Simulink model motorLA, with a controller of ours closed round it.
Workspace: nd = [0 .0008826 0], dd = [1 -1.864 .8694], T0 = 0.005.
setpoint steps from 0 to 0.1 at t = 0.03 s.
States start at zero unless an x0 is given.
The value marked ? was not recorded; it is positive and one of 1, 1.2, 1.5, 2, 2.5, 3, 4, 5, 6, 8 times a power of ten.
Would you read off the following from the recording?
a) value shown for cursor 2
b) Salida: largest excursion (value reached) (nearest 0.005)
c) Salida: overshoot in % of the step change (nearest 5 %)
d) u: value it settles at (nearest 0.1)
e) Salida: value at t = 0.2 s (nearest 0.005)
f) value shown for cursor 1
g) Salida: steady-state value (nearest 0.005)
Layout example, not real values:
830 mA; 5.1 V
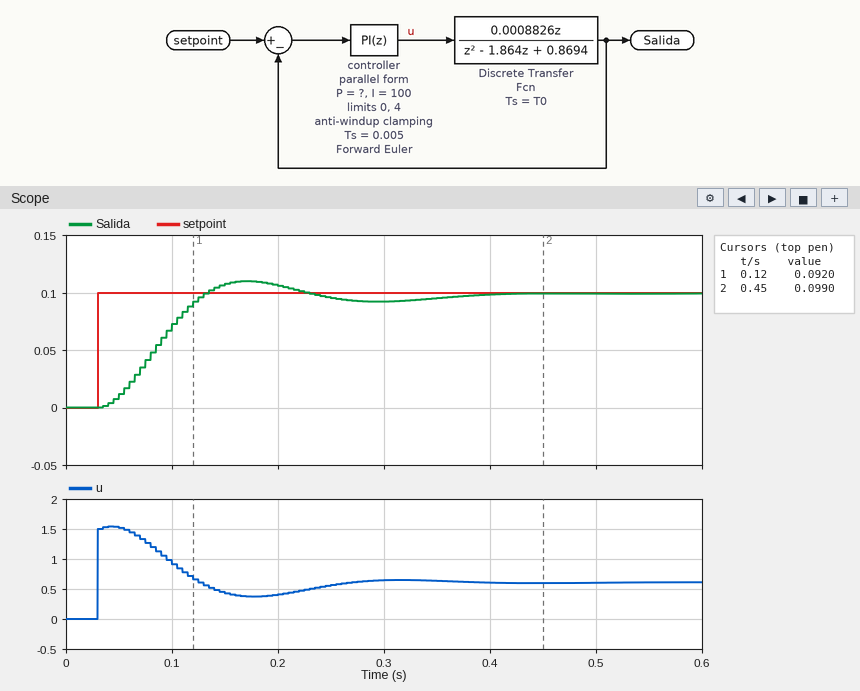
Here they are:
0.0990; 0.110; 10 %; 0.6; 0.105; 0.0920; 0.100
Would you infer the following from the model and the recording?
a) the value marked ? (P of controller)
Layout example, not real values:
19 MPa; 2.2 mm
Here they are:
15
